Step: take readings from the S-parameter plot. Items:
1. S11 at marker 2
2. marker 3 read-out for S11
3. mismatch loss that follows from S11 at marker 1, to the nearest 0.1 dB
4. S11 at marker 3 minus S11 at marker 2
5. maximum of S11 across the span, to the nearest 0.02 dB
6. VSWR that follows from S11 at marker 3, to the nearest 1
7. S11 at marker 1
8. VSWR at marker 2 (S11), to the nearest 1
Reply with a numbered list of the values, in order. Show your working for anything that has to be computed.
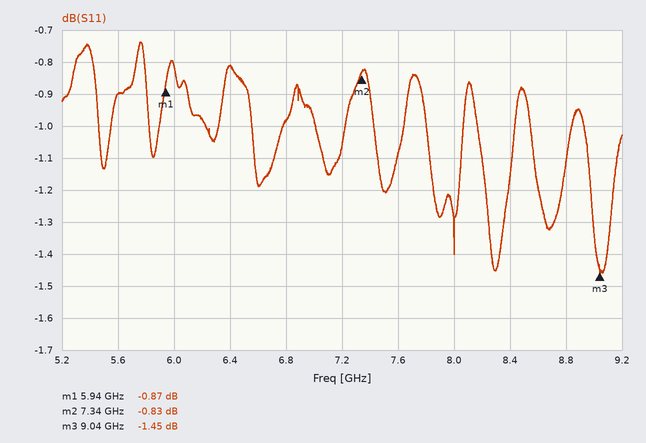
1. -0.83 dB
2. -1.45 dB
3. −10 log10(1 − 10^(-0.87/10)) ≈ 7.4 dB
4. -1.45 − (-0.83) = -0.62 dB
5. -0.74 dB
6. (1 + 0.8463)/(1 − 0.8463) ≈ 12
7. -0.87 dB
8. (1 + 0.9089)/(1 − 0.9089) ≈ 21
